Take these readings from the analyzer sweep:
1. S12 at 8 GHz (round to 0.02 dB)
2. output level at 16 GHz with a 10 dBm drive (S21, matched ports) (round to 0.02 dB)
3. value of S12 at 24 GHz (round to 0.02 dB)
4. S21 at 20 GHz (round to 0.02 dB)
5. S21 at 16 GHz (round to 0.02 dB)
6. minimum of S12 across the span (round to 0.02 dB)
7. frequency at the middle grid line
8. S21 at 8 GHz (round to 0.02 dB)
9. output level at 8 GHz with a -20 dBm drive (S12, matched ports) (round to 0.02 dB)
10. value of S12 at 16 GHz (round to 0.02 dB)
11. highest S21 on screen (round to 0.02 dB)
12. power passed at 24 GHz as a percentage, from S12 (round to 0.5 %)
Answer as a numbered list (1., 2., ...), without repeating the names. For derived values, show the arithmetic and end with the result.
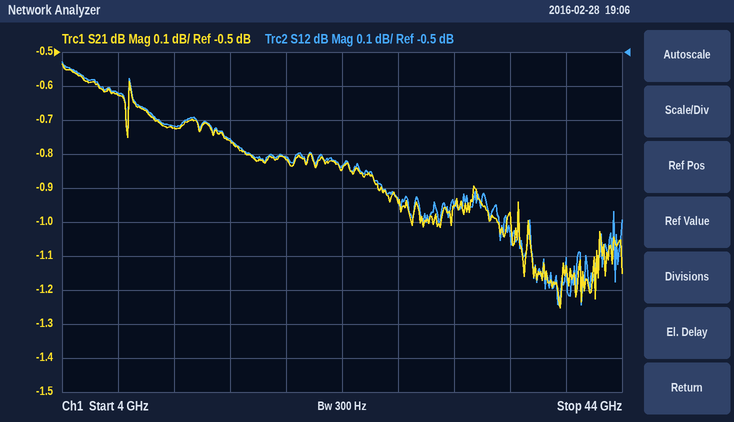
1. -0.62 dB
2. 10 dBm + (-0.76 dB) = 9.24 dBm
3. -0.84 dB
4. -0.82 dB
5. -0.76 dB
6. -1.24 dB
7. 24 GHz
8. -0.62 dB
9. -20 dBm + (-0.62 dB) = -20.62 dBm
10. -0.76 dB
11. -0.54 dB
12. 10^(-0.84/10) ≈ 82.4 %, so 82.5 % to the nearest 0.5 %
